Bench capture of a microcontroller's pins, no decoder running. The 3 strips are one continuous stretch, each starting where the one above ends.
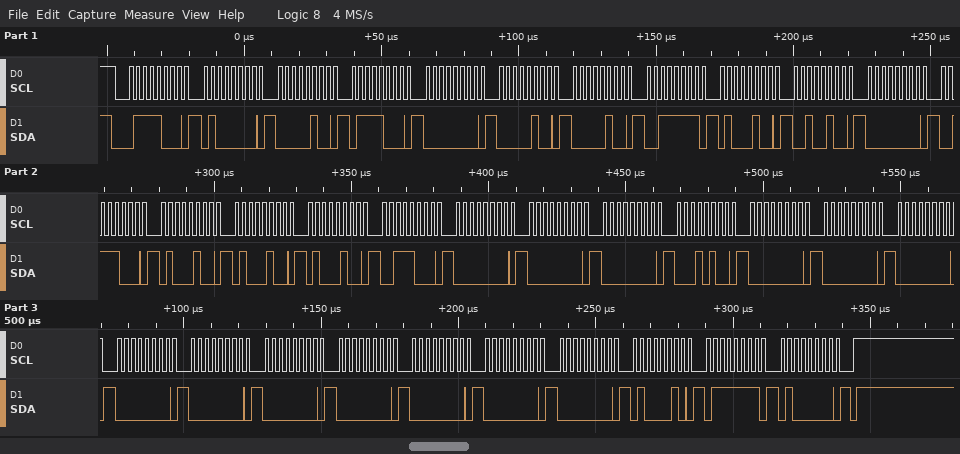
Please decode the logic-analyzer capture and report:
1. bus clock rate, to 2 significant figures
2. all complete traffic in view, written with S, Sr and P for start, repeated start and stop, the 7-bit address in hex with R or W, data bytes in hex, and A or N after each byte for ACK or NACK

400 kHz
S 3CW A 40 A 04 A 78 A 00 A 04 A 04 A 3F A 44 A 24 A 00 A 38 A 44 A 44 A 44 A 38 A 00 A 00 A 00 A 14 A 00 A 00 A 00 A 00 A 00 A 00 A 00 A 00 A 00 A 00 A 42 A 7F A 40 A P
